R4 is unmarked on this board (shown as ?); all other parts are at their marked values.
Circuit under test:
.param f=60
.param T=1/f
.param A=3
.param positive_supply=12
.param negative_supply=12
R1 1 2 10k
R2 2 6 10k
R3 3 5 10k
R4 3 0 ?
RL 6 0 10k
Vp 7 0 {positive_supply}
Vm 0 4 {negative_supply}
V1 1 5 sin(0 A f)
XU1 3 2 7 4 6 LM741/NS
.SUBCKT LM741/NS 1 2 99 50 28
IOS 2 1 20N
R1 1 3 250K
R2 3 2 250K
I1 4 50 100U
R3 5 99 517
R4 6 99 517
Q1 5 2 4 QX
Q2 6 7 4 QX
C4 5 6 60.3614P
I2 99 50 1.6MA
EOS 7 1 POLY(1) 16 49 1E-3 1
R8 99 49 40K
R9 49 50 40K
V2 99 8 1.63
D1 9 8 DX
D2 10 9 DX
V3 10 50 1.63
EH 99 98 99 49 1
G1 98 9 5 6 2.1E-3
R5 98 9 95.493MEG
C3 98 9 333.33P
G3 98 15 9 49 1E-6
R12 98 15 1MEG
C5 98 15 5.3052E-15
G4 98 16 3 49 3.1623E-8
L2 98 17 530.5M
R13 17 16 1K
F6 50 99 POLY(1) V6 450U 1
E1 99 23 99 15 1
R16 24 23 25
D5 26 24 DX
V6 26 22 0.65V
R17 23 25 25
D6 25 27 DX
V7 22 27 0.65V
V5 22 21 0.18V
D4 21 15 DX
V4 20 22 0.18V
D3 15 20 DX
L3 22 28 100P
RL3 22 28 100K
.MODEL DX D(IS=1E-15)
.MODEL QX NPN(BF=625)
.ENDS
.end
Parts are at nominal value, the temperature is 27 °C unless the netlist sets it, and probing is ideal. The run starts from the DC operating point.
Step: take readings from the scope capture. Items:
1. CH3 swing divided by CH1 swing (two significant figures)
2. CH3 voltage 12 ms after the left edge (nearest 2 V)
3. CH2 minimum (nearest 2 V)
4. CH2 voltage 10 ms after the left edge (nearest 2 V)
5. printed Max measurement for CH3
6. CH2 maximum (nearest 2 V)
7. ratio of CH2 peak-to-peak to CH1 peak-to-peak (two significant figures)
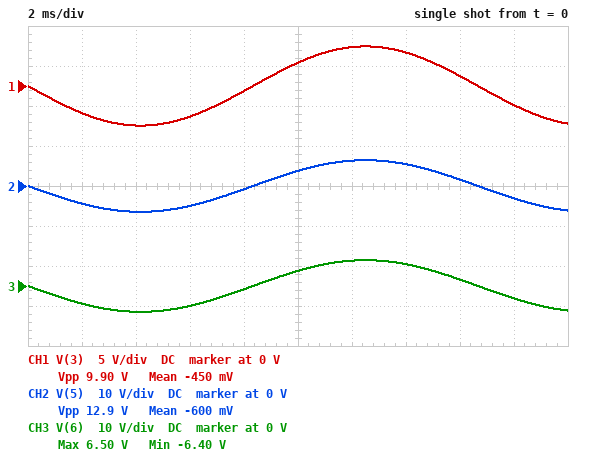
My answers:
1.3
6 V
-6 V
4 V
6.50 V
6 V
1.3
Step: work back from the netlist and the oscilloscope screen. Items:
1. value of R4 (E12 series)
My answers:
33 kΩ
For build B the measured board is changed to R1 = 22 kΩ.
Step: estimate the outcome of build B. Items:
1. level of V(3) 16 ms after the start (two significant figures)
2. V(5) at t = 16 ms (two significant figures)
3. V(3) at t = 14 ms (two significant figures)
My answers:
770 mV
1.0 V
2.6 V
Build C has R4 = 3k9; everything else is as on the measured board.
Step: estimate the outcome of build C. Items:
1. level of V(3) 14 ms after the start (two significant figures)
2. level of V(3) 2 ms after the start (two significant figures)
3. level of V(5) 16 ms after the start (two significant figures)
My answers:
490 mV
-400 mV
520 mV
